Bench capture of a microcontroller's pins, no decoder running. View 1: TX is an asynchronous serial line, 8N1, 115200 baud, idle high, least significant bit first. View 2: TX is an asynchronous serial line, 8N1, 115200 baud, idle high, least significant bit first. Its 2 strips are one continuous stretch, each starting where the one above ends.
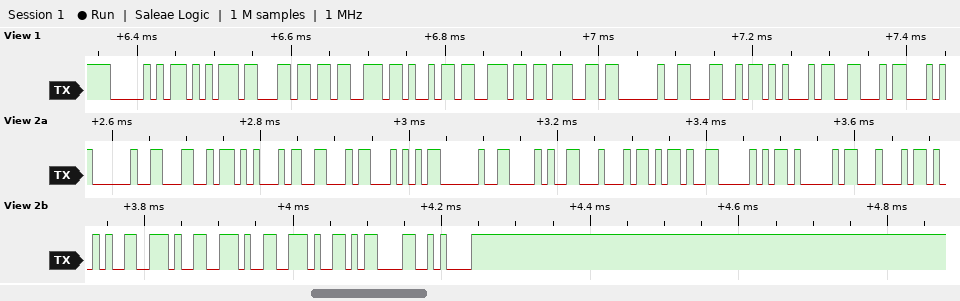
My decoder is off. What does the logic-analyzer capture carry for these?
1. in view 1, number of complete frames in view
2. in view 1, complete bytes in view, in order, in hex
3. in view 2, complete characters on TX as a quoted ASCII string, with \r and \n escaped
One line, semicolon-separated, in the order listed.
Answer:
11; 50 75 6C 73 69 6E 67 20 4C 45 46; " LEFT (D-PAD)...\r\n"
